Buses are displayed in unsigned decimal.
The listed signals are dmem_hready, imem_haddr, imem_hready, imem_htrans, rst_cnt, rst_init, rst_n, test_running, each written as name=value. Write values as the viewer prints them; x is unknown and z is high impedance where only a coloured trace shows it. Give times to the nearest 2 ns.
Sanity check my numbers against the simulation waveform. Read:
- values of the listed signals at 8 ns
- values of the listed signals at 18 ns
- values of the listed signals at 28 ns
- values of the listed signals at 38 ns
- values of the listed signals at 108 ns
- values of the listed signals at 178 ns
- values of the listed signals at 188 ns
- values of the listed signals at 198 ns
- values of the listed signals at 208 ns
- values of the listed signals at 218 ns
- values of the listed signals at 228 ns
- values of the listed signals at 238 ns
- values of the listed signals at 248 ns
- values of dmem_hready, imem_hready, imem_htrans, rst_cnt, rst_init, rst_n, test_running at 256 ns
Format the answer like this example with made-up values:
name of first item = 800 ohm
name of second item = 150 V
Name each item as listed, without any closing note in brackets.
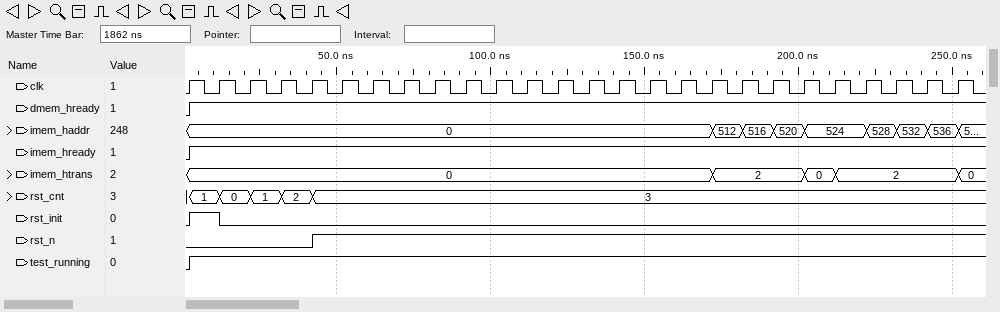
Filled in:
values of the listed signals at 8 ns = dmem_hready=1, imem_haddr=0, imem_hready=1, imem_htrans=0, rst_cnt=1, rst_init=1, rst_n=0, test_running=1
values of the listed signals at 18 ns = dmem_hready=1, imem_haddr=0, imem_hready=1, imem_htrans=0, rst_cnt=0, rst_init=0, rst_n=0, test_running=1
values of the listed signals at 28 ns = dmem_hready=1, imem_haddr=0, imem_hready=1, imem_htrans=0, rst_cnt=1, rst_init=0, rst_n=0, test_running=1
values of the listed signals at 38 ns = dmem_hready=1, imem_haddr=0, imem_hready=1, imem_htrans=0, rst_cnt=2, rst_init=0, rst_n=0, test_running=1
values of the listed signals at 108 ns = dmem_hready=1, imem_haddr=0, imem_hready=1, imem_htrans=0, rst_cnt=3, rst_init=0, rst_n=1, test_running=1
values of the listed signals at 178 ns = dmem_hready=1, imem_haddr=512, imem_hready=1, imem_htrans=2, rst_cnt=3, rst_init=0, rst_n=1, test_running=1
values of the listed signals at 188 ns = dmem_hready=1, imem_haddr=516, imem_hready=1, imem_htrans=2, rst_cnt=3, rst_init=0, rst_n=1, test_running=1
values of the listed signals at 198 ns = dmem_hready=1, imem_haddr=520, imem_hready=1, imem_htrans=2, rst_cnt=3, rst_init=0, rst_n=1, test_running=1
values of the listed signals at 208 ns = dmem_hready=1, imem_haddr=524, imem_hready=1, imem_htrans=0, rst_cnt=3, rst_init=0, rst_n=1, test_running=1
values of the listed signals at 218 ns = dmem_hready=1, imem_haddr=524, imem_hready=1, imem_htrans=2, rst_cnt=3, rst_init=0, rst_n=1, test_running=1
values of the listed signals at 228 ns = dmem_hready=1, imem_haddr=528, imem_hready=1, imem_htrans=2, rst_cnt=3, rst_init=0, rst_n=1, test_running=1
values of the listed signals at 238 ns = dmem_hready=1, imem_haddr=532, imem_hready=1, imem_htrans=2, rst_cnt=3, rst_init=0, rst_n=1, test_running=1
values of the listed signals at 248 ns = dmem_hready=1, imem_haddr=536, imem_hready=1, imem_htrans=2, rst_cnt=3, rst_init=0, rst_n=1, test_running=1
values of dmem_hready, imem_hready, imem_htrans, rst_cnt, rst_init, rst_n, test_running at 256 ns = dmem_hready=1, imem_hready=1, imem_htrans=0, rst_cnt=3, rst_init=0, rst_n=1, test_running=1
